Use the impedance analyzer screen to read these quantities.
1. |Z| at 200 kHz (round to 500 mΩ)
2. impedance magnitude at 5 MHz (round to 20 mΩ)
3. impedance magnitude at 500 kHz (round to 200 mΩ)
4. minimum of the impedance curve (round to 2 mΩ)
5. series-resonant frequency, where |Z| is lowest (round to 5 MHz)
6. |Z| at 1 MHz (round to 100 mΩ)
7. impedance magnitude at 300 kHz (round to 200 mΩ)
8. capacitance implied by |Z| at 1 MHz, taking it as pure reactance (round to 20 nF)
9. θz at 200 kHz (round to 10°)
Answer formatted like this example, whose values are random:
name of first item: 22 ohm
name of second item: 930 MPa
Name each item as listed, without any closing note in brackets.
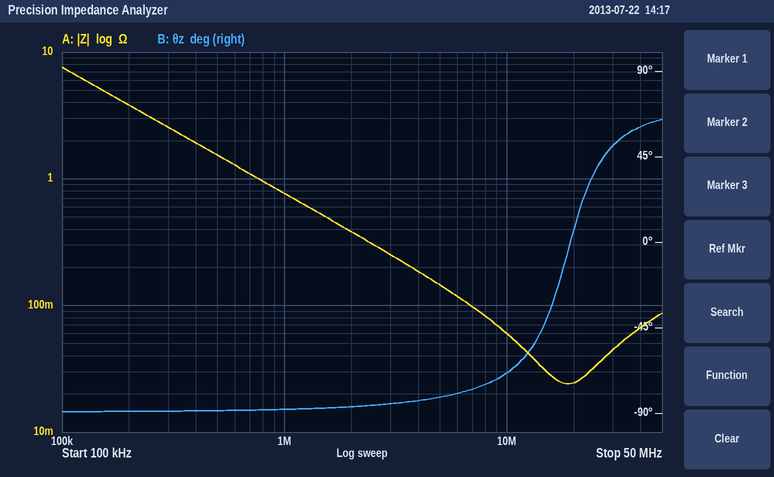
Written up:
|Z| at 200 kHz: 4.0 Ω
impedance magnitude at 5 MHz: 140 mΩ
impedance magnitude at 500 kHz: 1.6 Ω
minimum of the impedance curve: 24 mΩ
series-resonant frequency, where |Z| is lowest: 20 MHz
|Z| at 1 MHz: 800 mΩ
impedance magnitude at 300 kHz: 2.6 Ω
capacitance implied by |Z| at 1 MHz, taking it as pure reactance: 200 nF
θz at 200 kHz: -90°
